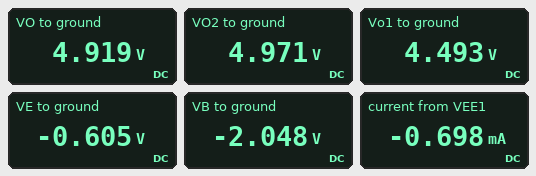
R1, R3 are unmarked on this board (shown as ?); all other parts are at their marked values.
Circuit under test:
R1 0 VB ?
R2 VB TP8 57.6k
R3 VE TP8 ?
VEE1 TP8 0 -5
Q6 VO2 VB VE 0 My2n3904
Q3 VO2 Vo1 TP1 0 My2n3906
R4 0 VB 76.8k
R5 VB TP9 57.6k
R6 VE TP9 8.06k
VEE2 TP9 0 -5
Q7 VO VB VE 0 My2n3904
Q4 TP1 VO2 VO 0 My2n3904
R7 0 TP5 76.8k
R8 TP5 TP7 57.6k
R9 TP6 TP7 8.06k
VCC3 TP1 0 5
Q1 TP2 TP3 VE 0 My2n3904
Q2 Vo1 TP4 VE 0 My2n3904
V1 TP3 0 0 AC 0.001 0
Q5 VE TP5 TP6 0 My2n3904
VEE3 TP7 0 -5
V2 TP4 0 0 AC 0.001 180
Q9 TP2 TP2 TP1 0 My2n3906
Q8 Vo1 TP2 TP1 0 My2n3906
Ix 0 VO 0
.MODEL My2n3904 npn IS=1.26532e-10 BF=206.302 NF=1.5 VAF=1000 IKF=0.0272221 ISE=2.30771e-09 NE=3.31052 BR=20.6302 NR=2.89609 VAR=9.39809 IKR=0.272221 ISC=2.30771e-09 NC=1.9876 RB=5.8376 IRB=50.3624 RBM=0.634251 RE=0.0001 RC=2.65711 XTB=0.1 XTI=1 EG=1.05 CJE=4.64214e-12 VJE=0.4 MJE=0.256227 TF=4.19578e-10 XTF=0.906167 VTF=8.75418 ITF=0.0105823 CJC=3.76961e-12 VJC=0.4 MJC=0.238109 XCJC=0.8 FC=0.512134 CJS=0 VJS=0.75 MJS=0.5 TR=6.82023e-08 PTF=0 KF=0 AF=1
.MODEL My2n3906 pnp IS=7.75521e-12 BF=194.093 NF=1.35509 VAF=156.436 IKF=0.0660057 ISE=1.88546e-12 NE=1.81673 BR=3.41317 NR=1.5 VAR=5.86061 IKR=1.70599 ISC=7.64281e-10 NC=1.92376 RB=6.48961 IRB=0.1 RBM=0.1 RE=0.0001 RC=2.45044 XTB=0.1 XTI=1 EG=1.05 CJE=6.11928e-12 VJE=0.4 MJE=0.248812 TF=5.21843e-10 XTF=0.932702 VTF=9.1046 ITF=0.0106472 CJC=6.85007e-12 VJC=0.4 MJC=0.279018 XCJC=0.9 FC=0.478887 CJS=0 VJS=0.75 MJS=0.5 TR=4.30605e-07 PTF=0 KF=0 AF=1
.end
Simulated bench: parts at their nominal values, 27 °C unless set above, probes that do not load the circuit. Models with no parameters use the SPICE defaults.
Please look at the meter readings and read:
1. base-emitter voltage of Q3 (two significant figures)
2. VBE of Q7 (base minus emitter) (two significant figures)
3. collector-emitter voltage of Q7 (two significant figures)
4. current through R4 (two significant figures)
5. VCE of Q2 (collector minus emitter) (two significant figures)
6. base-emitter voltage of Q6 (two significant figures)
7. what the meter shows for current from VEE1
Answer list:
-510 mV
-1.4 V
5.5 V
27 µA
5.1 V
-1.4 V
-0.698 mA
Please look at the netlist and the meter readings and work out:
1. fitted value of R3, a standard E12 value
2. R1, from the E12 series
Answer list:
6.8 kΩ
27 kΩ
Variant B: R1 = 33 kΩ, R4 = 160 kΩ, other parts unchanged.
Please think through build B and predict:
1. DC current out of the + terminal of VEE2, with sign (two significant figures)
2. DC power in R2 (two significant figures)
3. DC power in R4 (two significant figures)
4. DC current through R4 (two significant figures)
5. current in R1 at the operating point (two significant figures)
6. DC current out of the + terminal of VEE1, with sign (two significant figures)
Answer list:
-590 µA
110 µW
37 µW
15 µA
74 µA
-690 µA
